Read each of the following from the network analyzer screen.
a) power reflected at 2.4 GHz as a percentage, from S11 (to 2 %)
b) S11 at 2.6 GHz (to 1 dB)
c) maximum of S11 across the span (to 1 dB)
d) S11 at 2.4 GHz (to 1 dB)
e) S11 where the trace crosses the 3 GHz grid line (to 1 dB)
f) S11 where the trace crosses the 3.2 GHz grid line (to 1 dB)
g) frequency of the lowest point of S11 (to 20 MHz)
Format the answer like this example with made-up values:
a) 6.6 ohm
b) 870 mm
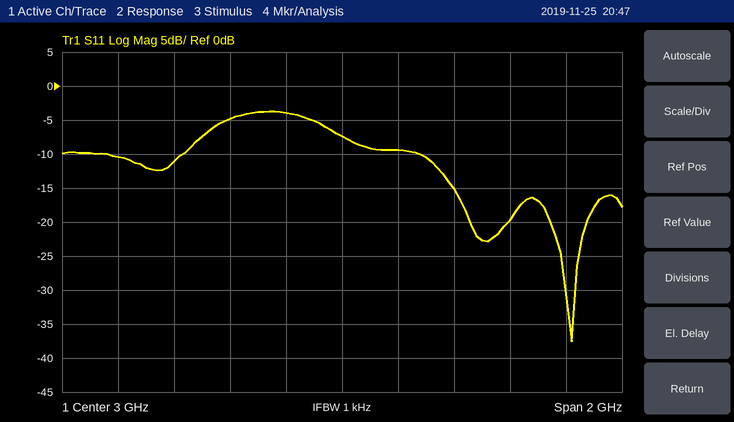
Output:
a) 8 %
b) -5 dB
c) -4 dB
d) -11 dB
e) -7 dB
f) -9 dB
g) 3.82 GHz
